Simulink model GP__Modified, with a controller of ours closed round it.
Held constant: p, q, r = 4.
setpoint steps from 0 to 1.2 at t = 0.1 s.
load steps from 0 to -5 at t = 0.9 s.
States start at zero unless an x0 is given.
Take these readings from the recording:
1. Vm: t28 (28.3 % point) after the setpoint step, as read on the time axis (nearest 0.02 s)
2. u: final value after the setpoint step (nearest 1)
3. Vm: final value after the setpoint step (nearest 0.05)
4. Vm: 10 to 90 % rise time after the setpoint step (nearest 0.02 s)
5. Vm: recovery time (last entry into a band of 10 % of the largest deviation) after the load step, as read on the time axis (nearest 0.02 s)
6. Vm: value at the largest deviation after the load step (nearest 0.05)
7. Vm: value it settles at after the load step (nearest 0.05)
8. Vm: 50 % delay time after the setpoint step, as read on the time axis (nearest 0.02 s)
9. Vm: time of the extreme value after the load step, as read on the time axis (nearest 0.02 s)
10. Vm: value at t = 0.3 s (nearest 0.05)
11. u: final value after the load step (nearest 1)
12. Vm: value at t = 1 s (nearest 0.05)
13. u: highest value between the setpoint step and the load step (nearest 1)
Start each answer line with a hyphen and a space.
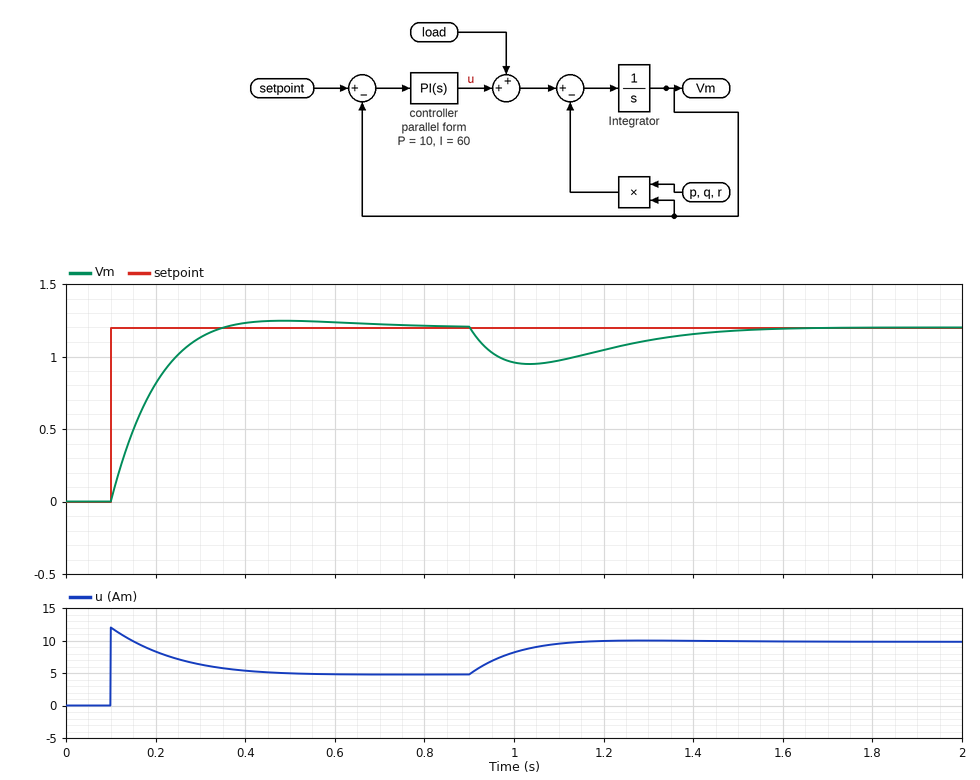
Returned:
- 0.14 s
- 5
- 1.20
- 0.16 s
- 1.48 s
- 0.95
- 1.20
- 0.16 s
- 1.04 s
- 1.15
- 10
- 0.95
- 12
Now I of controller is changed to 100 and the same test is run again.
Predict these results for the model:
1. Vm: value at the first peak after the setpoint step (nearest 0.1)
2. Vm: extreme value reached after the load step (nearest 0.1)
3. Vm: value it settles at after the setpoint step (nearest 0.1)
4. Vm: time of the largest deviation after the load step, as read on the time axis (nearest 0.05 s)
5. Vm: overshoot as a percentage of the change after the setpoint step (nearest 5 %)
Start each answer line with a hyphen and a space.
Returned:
- 1.3
- 1.0
- 1.2
- 1.00 s
- 10 %
